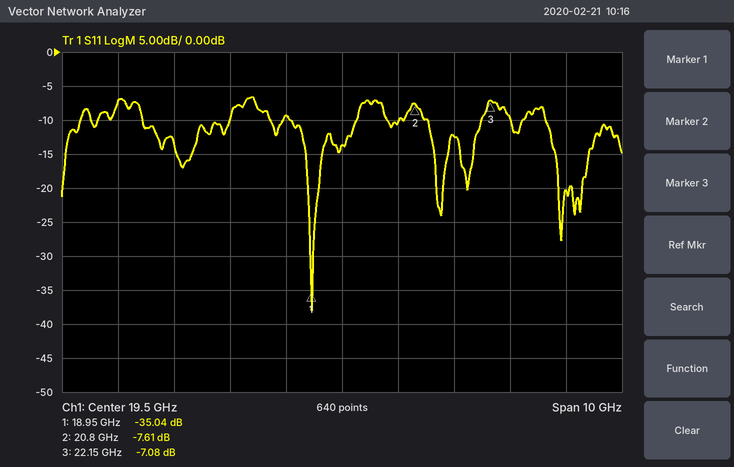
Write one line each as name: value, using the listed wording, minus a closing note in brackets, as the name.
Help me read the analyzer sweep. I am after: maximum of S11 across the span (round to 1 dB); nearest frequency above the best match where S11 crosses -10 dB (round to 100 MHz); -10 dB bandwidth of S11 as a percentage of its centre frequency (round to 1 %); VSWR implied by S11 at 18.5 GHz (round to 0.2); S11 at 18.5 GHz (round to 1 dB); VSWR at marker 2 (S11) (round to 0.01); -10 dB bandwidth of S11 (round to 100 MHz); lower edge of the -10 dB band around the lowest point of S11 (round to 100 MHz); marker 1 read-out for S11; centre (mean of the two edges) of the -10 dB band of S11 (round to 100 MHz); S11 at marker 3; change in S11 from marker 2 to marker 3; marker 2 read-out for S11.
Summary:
maximum of S11 across the span: -7 dB
nearest frequency above the best match where S11 crosses -10 dB: 19.8 GHz
-10 dB bandwidth of S11 as a percentage of its centre frequency: 6 %
VSWR implied by S11 at 18.5 GHz: 2.0
S11 at 18.5 GHz: -9 dB
VSWR at marker 2 (S11): 2.43
-10 dB bandwidth of S11: 1.2 GHz
lower edge of the -10 dB band around the lowest point of S11: 18.6 GHz
marker 1 read-out for S11: -35.04 dB
centre (mean of the two edges) of the -10 dB band of S11: 19.2 GHz
S11 at marker 3: -7.08 dB
change in S11 from marker 2 to marker 3: 0.53 dB
marker 2 read-out for S11: -7.61 dB
